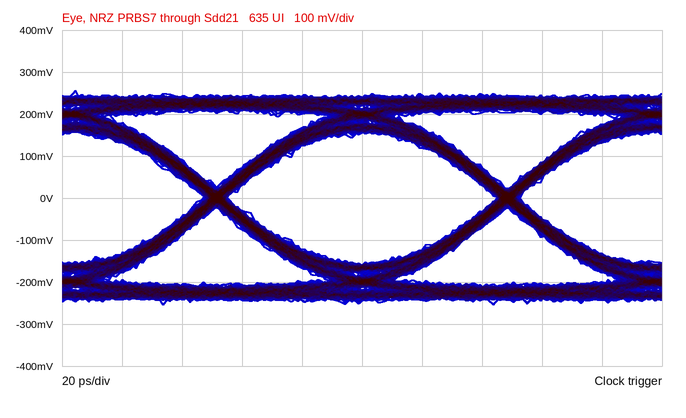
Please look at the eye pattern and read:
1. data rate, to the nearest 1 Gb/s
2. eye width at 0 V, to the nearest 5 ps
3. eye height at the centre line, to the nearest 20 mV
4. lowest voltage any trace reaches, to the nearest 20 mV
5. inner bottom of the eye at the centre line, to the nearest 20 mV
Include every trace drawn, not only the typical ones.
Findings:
10 Gb/s
90 ps
320 mV
-260 mV
-160 mV
